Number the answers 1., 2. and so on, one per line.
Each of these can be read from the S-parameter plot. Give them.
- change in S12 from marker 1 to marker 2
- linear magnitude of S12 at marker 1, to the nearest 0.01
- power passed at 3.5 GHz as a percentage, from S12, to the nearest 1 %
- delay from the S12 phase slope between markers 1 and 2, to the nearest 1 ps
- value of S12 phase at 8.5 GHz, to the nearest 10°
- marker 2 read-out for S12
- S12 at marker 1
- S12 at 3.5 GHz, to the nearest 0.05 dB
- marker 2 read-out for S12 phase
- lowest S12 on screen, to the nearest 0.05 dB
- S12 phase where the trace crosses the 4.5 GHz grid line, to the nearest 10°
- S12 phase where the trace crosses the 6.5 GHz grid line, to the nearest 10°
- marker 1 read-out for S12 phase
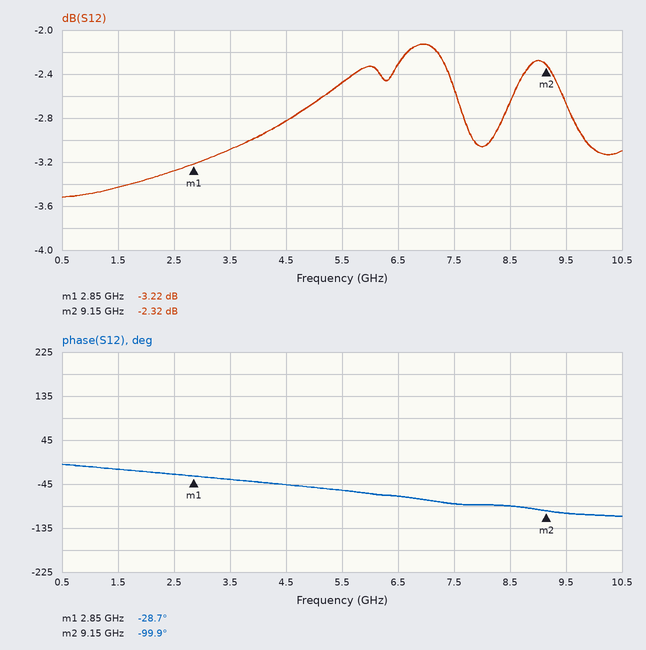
1. 0.90 dB
2. 0.69
3. 49 %
4. 31 ps
5. -90°
6. -2.32 dB
7. -3.22 dB
8. -3.10 dB
9. -99.9°
10. -3.50 dB
11. -50°
12. -70°
13. -28.7°
